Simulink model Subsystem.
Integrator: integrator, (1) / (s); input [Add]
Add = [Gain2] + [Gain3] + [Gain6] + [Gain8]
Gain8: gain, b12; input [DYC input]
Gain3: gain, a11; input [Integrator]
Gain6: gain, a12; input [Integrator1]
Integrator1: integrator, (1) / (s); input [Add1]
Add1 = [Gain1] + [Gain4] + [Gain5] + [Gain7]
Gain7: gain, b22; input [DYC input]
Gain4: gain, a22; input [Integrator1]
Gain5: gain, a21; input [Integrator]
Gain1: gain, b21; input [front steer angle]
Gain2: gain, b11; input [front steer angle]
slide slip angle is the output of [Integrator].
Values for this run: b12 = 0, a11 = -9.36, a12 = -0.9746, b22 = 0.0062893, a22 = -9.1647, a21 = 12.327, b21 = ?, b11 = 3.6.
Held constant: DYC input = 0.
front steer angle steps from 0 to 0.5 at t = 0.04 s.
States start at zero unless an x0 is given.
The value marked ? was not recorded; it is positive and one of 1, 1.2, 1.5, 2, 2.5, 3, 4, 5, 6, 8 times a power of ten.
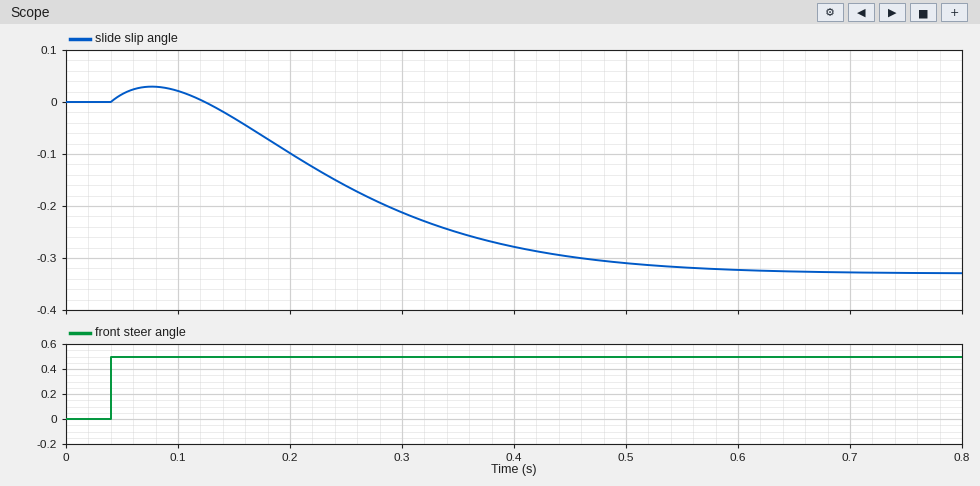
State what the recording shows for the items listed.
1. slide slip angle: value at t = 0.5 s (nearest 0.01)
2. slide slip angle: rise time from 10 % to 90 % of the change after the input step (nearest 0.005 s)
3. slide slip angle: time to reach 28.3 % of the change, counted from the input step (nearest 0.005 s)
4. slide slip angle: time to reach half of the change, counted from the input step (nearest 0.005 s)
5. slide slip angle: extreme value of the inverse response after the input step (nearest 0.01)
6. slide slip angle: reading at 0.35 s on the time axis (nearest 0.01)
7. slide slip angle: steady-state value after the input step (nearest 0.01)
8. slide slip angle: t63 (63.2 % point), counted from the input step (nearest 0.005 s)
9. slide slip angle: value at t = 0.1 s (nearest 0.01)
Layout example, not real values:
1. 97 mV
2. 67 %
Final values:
1. -0.31
2. 0.295 s
3. 0.155 s
4. 0.215 s
5. 0.03
6. -0.25
7. -0.33
8. 0.255 s
9. 0.02
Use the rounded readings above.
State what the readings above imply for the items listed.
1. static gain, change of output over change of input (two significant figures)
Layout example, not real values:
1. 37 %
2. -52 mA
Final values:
1. -0.66
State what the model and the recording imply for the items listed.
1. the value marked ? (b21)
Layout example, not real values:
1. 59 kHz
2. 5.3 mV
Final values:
1. 100
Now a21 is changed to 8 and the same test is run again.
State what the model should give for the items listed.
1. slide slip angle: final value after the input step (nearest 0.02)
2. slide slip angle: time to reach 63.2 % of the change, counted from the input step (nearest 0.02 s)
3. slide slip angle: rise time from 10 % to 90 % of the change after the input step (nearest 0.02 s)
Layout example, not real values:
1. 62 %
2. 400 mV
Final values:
1. -0.34
2. 0.26 s
3. 0.32 s
